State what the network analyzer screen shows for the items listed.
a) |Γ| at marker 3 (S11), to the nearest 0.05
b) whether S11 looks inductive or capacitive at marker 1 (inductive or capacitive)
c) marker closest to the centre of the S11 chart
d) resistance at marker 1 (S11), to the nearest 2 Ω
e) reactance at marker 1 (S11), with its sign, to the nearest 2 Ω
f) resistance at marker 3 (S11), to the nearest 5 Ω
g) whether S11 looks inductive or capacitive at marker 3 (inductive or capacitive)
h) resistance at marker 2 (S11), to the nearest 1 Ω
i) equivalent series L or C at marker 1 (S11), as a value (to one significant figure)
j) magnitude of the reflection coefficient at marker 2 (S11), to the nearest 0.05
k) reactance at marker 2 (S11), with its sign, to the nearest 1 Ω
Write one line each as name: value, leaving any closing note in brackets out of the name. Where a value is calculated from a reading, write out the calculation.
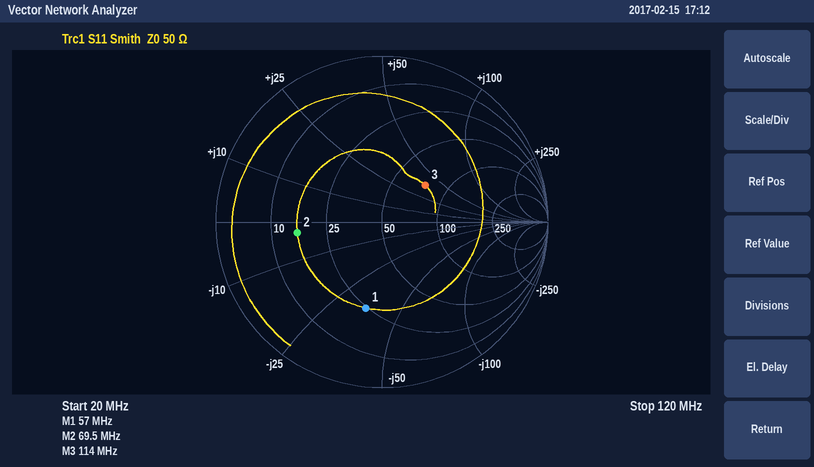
|Γ| at marker 3 (S11), to the nearest 0.05: 0.35
whether S11 looks inductive or capacitive at marker 1: capacitive
marker closest to the centre of the S11 chart: marker 3
resistance at marker 1 (S11), to the nearest 2 Ω: 24 Ω
reactance at marker 1 (S11), with its sign, to the nearest 2 Ω: -36 Ω
resistance at marker 3 (S11), to the nearest 5 Ω: 75 Ω
whether S11 looks inductive or capacitive at marker 3: inductive
resistance at marker 2 (S11), to the nearest 1 Ω: 16 Ω
equivalent series L or C at marker 1 (S11), as a value: C = 1/(2π × 57 MHz × 36 Ω) ≈ 77.6 pF, so 80 pF to one significant figure
magnitude of the reflection coefficient at marker 2 (S11), to the nearest 0.05: 0.50
reactance at marker 2 (S11), with its sign, to the nearest 1 Ω: -3 Ω
